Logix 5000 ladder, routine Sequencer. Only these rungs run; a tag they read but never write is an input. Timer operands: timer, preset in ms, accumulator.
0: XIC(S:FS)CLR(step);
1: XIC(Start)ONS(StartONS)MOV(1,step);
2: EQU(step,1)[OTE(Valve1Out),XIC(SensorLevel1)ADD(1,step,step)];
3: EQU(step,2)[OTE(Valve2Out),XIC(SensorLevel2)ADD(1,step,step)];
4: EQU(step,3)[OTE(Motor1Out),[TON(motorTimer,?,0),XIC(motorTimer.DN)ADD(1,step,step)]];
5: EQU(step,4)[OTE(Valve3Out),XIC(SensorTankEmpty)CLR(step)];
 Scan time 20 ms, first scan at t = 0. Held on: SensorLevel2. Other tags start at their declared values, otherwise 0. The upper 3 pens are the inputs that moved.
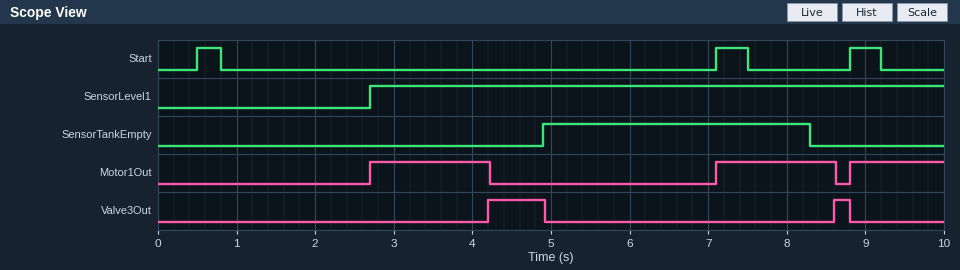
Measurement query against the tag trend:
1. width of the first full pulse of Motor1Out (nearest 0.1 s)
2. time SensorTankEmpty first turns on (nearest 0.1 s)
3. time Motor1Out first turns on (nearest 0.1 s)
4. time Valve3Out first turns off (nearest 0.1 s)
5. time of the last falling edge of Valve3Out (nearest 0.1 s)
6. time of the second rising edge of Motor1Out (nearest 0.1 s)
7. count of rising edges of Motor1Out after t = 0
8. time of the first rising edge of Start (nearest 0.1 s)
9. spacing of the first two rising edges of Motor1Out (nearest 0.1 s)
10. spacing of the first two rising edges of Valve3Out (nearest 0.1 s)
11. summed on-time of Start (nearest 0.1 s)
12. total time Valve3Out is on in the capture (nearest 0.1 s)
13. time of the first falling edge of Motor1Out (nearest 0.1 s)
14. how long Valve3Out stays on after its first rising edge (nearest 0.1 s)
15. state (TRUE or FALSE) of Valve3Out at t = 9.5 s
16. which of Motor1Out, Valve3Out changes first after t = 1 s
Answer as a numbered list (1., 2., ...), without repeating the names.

1. 1.5 s
2. 4.9 s
3. 2.7 s
4. 4.9 s
5. 8.8 s
6. 7.1 s
7. 3
8. 0.5 s
9. 4.4 s
10. 4.4 s
11. 1.1 s
12. 0.9 s
13. 4.2 s
14. 0.7 s
15. FALSE
16. Motor1Out
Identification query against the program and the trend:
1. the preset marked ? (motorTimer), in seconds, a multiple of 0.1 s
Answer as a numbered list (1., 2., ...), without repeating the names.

1. 1.5 s
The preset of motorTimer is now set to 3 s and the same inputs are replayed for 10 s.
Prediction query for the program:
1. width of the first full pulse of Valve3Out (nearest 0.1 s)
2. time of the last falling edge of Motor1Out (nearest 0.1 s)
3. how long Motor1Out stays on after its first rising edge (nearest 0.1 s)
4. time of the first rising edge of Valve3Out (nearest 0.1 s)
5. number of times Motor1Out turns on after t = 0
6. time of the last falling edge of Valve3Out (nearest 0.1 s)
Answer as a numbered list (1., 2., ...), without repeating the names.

1. 0.0 s
2. 5.7 s
3. 3.0 s
4. 5.7 s
5. 2
6. 5.7 s
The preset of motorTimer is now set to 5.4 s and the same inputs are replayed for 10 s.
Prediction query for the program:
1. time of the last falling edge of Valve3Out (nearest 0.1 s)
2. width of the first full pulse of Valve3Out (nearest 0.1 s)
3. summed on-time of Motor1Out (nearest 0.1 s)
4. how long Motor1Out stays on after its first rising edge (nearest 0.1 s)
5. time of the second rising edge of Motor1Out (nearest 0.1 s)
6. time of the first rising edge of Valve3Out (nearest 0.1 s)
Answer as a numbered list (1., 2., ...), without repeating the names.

1. 8.1 s
2. 0.0 s
3. 6.6 s
4. 5.4 s
5. 8.8 s
6. 8.1 s
